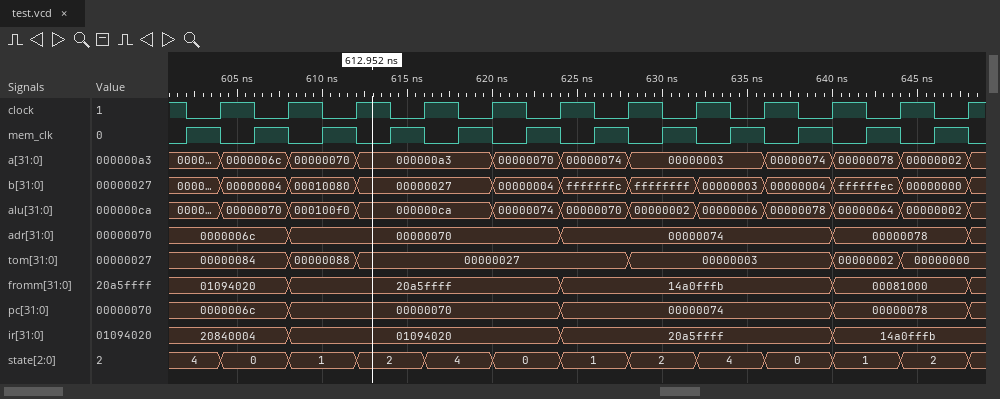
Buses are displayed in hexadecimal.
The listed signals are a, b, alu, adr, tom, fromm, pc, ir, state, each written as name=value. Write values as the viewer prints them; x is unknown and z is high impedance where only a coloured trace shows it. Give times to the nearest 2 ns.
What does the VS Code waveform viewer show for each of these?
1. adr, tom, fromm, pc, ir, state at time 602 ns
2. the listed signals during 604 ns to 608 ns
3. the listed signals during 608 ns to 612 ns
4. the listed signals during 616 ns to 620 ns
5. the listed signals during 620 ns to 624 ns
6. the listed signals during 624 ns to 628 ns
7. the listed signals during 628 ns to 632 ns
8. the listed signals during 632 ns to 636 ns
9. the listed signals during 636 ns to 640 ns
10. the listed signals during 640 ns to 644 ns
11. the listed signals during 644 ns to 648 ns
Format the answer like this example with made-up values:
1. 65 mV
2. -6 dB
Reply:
1. adr=0000006c, tom=00000084, fromm=01094020, pc=0000006c, ir=20840004, state=4
2. a=0000006c, b=00000004, alu=00000070, adr=0000006c, tom=00000084, fromm=01094020, pc=0000006c, ir=20840004, state=0
3. a=00000070, b=00010080, alu=000100f0, adr=00000070, tom=00000088, fromm=20a5ffff, pc=00000070, ir=01094020, state=1
4. a=000000a3, b=00000027, alu=000000ca, adr=00000070, tom=00000027, fromm=20a5ffff, pc=00000070, ir=01094020, state=4
5. a=00000070, b=00000004, alu=00000074, adr=00000070, tom=00000027, fromm=20a5ffff, pc=00000070, ir=01094020, state=0
6. a=00000074, b=fffffffc, alu=00000070, adr=00000074, tom=00000027, fromm=14a0fffb, pc=00000074, ir=20a5ffff, state=1
7. a=00000003, b=ffffffff, alu=00000002, adr=00000074, tom=00000003, fromm=14a0fffb, pc=00000074, ir=20a5ffff, state=2
8. a=00000003, b=00000003, alu=00000006, adr=00000074, tom=00000003, fromm=14a0fffb, pc=00000074, ir=20a5ffff, state=4
9. a=00000074, b=00000004, alu=00000078, adr=00000074, tom=00000003, fromm=14a0fffb, pc=00000074, ir=20a5ffff, state=0
10. a=00000078, b=ffffffec, alu=00000064, adr=00000078, tom=00000002, fromm=00081000, pc=00000078, ir=14a0fffb, state=1
11. a=00000002, b=00000000, alu=00000002, adr=00000078, tom=00000000, fromm=00081000, pc=00000078, ir=14a0fffb, state=2
